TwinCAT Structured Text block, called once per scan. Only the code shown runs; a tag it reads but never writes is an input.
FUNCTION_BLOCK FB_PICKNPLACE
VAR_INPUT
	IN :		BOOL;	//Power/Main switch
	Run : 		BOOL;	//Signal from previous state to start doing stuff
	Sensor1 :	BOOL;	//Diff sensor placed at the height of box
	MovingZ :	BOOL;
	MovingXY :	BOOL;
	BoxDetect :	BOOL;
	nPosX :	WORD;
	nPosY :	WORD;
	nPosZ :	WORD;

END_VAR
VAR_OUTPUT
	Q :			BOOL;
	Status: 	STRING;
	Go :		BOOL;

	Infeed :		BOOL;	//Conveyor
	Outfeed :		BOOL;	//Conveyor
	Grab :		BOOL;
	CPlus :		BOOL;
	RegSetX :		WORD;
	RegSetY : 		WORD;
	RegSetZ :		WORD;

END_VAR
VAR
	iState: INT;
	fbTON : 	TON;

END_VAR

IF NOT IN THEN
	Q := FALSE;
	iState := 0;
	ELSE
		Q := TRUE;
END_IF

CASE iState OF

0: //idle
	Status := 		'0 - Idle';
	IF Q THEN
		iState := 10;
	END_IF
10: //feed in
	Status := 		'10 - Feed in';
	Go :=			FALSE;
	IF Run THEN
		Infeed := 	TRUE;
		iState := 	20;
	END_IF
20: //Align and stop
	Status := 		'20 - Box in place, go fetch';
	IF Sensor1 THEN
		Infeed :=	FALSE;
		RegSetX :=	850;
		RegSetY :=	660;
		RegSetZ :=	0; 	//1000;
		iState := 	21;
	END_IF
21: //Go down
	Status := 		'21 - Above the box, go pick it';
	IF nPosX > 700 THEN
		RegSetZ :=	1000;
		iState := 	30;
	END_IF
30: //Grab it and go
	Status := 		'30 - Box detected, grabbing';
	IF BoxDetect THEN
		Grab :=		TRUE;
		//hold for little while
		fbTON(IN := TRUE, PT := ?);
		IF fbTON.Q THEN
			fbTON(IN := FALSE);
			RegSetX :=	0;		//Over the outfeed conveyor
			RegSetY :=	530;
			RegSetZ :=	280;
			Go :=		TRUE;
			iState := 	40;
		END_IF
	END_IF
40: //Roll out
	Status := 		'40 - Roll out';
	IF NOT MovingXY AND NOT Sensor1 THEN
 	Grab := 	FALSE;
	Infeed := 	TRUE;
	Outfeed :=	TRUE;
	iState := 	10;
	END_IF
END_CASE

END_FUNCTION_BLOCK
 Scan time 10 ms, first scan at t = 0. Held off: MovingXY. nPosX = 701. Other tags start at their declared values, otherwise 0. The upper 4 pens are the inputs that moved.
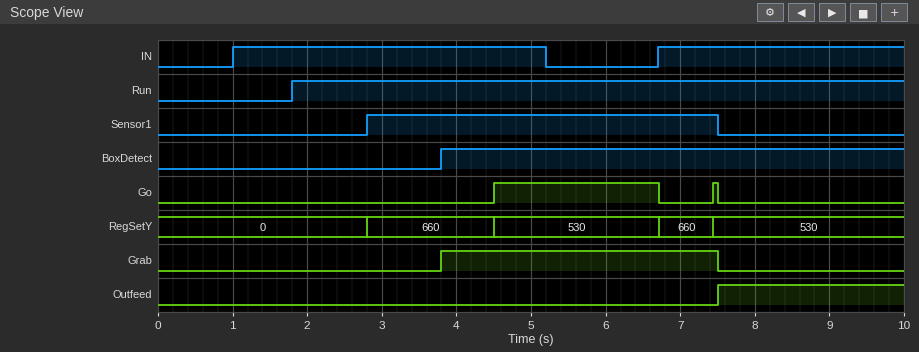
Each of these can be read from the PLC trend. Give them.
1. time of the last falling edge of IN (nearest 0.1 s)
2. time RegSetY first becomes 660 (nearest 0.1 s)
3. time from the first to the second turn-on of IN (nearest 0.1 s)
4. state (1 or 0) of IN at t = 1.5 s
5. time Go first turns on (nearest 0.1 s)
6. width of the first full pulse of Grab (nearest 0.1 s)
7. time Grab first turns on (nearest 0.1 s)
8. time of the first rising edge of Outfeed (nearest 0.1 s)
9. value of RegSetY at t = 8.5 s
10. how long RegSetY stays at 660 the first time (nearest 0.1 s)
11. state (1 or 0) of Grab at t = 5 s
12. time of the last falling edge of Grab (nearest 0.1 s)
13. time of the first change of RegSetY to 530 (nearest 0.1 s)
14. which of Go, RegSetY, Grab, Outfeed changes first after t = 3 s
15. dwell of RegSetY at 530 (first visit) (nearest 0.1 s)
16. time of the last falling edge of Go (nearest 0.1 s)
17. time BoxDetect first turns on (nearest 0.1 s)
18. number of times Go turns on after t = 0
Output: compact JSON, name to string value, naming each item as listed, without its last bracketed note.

{"time of the last falling edge of IN": "5.2 s", "time RegSetY first becomes 660": "2.8 s", "time from the first to the second turn-on of IN": "5.7 s", "state (1 or 0) of IN at t = 1.5 s": "1", "time Go first turns on": "4.5 s", "width of the first full pulse of Grab": "3.7 s", "time Grab first turns on": "3.8 s", "time of the first rising edge of Outfeed": "7.5 s", "value of RegSetY at t = 8.5 s": "530", "how long RegSetY stays at 660 the first time": "1.7 s", "state (1 or 0) of Grab at t = 5 s": "1", "time of the last falling edge of Grab": "7.5 s", "time of the first change of RegSetY to 530": "4.5 s", "which of Go, RegSetY, Grab, Outfeed changes first after t = 3 s": "Grab", "dwell of RegSetY at 530 (first visit)": "2.2 s", "time of the last falling edge of Go": "7.5 s", "time BoxDetect first turns on": "3.8 s", "number of times Go turns on after t = 0": "2"}
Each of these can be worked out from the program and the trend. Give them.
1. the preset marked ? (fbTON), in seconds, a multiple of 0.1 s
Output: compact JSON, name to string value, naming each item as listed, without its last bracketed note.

{"the preset marked ? (fbTON), in seconds, a multiple of 0.1 s": "0.7 s"}
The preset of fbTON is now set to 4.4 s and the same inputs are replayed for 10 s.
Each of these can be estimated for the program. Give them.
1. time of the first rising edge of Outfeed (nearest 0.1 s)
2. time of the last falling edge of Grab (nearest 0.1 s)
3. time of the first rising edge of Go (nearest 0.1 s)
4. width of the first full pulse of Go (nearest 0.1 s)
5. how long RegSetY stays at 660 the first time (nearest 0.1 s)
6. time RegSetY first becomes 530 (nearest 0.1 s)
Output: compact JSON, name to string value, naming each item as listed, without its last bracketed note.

{"time of the first rising edge of Outfeed": "8.2 s", "time of the last falling edge of Grab": "8.2 s", "time of the first rising edge of Go": "8.2 s", "width of the first full pulse of Go": "0.0 s", "how long RegSetY stays at 660 the first time": "5.4 s", "time RegSetY first becomes 530": "8.2 s"}
